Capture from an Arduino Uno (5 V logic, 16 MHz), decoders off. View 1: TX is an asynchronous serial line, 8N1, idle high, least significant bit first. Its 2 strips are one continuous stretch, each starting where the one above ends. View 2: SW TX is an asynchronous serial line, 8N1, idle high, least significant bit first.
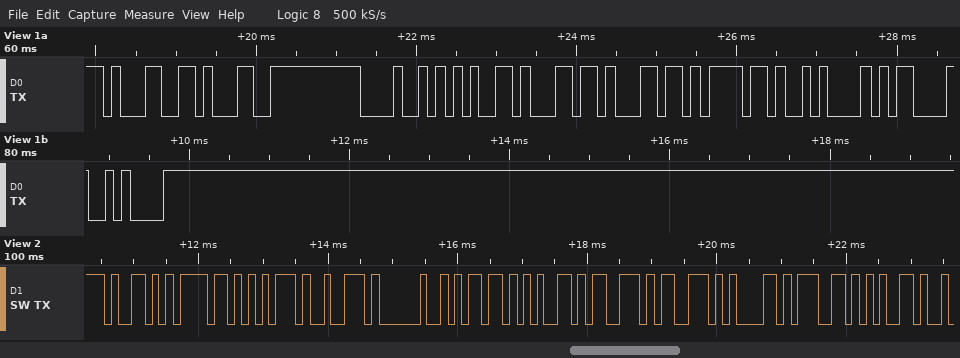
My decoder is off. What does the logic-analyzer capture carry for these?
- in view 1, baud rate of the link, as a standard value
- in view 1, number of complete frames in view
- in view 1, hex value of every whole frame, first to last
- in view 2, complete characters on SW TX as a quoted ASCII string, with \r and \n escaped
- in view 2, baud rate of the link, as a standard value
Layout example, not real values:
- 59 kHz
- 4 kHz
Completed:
- 9600 baud
- 10
- 0x31 0x31 0x48 0x65 0x6C 0x6C 0x6F 0x0A 0x0D 0x0A
- "Your message"
- 9600 baud
